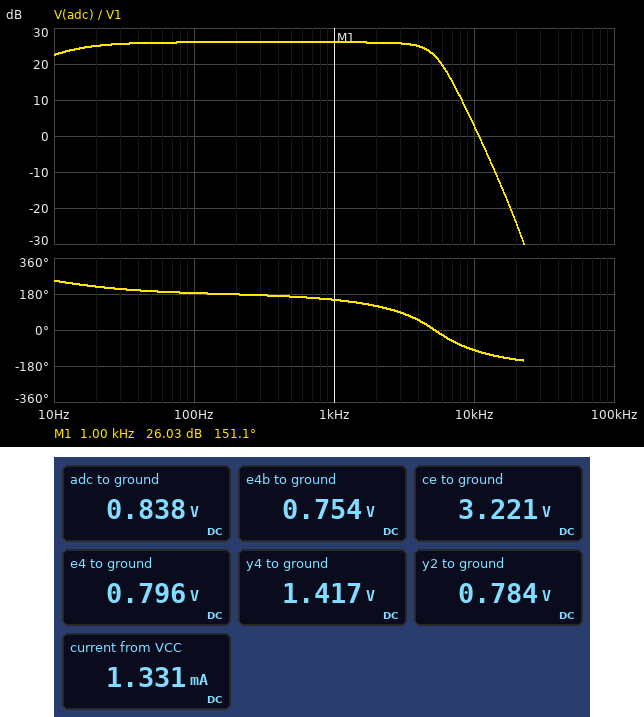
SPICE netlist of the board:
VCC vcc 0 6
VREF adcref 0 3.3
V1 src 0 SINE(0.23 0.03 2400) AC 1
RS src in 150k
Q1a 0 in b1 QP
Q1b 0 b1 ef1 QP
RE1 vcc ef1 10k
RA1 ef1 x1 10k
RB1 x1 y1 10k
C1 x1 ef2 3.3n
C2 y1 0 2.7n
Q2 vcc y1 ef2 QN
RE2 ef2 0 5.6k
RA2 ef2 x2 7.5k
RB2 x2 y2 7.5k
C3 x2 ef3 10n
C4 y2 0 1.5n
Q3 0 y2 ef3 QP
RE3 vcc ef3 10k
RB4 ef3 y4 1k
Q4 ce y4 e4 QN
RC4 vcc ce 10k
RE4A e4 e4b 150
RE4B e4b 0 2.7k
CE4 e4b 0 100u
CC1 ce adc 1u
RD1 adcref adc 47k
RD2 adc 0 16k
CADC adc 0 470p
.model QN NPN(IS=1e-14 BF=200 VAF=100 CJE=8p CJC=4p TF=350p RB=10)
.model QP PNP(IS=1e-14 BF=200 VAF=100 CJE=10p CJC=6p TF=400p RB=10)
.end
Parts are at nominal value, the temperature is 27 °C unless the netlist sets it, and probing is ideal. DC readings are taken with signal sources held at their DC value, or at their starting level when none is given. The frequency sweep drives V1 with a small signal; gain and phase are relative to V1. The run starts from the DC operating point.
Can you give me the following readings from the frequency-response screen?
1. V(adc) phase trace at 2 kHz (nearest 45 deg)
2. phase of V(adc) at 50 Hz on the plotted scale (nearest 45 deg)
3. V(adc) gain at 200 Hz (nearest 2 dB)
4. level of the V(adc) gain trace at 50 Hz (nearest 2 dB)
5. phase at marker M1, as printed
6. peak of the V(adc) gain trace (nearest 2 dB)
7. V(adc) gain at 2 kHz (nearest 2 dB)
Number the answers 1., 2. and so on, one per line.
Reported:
1. 135 deg
2. 180 deg
3. 26 dB
4. 26 dB
5. 151.1 deg
6. 26 dB
7. 26 dB
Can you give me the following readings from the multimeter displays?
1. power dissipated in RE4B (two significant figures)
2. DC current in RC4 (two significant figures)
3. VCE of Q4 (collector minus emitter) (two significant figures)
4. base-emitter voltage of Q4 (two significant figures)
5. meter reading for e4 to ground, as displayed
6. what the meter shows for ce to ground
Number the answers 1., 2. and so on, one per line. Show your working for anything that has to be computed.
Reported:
1. (754 mV)^2 / 2.7 kΩ = 210 µW
2. (6 V - 3.221 V) / 10 kΩ = 280 µA
3. 3.221 V - 796 mV = 2.4 V
4. 1.417 V - 796 mV = 620 mV
5. 0.796 V
6. 3.221 V
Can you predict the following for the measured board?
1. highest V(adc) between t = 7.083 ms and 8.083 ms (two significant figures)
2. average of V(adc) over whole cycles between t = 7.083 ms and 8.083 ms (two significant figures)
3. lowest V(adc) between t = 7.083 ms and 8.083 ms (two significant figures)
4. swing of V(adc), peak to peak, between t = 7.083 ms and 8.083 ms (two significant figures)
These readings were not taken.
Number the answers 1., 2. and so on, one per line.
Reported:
1. 1.4 V
2. 830 mV
3. 220 mV
4. 1.2 V
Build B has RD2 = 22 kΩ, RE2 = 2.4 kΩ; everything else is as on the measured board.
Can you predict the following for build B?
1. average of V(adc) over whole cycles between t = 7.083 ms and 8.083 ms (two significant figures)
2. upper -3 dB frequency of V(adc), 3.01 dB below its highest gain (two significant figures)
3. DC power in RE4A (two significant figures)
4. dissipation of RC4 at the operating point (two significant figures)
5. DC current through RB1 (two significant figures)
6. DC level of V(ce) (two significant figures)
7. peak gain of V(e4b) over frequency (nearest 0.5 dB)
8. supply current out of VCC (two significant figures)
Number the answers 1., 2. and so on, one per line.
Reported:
1. 1.0 V
2. 5.1 kHz
3. 11 µW
4. 710 µW
5. 1.4 µA
6. 3.3 V
7. -1.5 dB
8. 1.5 mA
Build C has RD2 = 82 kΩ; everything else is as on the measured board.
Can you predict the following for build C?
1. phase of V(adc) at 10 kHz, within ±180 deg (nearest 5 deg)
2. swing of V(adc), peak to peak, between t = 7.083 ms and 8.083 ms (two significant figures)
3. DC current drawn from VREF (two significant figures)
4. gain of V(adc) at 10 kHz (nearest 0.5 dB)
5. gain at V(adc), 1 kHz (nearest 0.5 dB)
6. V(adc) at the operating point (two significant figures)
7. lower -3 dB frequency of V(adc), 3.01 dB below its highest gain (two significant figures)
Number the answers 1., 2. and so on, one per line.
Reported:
1. -105 deg
2. 1.6 V
3. 26 µA
4. 5.5 dB
5. 29.0 dB
6. 2.1 V
7. 8.6 Hz
